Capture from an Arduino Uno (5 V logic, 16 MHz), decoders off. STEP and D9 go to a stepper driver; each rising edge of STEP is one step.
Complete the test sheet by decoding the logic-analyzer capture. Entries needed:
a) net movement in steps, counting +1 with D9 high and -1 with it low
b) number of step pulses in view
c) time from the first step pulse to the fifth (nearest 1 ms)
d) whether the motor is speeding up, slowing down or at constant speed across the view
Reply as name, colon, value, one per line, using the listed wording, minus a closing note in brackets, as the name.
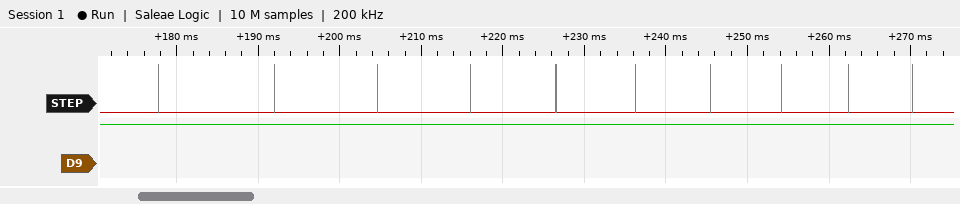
net movement in steps, counting +1 with D9 high and -1 with it low: +10
number of step pulses in view: 10
time from the first step pulse to the fifth: 49 ms
whether the motor is speeding up, slowing down or at constant speed across the view: speeding up
